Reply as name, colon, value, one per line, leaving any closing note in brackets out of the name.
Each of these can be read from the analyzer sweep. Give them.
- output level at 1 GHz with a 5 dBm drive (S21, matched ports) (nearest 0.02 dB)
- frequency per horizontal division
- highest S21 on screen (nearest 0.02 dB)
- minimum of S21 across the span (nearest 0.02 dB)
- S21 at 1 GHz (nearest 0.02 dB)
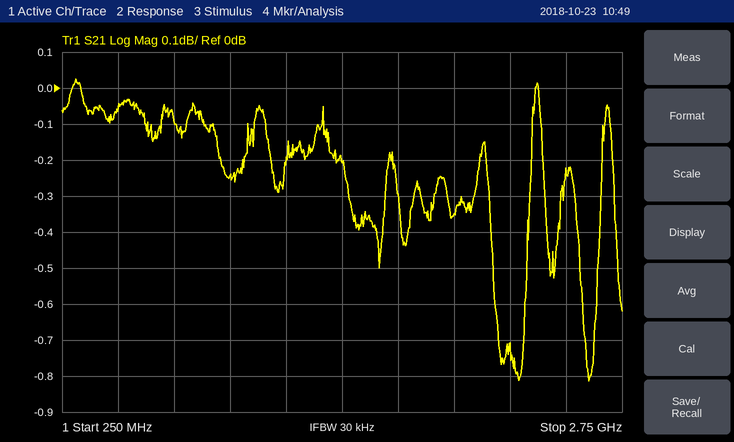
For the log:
output level at 1 GHz with a 5 dBm drive (S21, matched ports): 4.76 dBm
frequency per horizontal division: 250 MHz
highest S21 on screen: 0.02 dB
minimum of S21 across the span: -0.82 dB
S21 at 1 GHz: -0.24 dB
